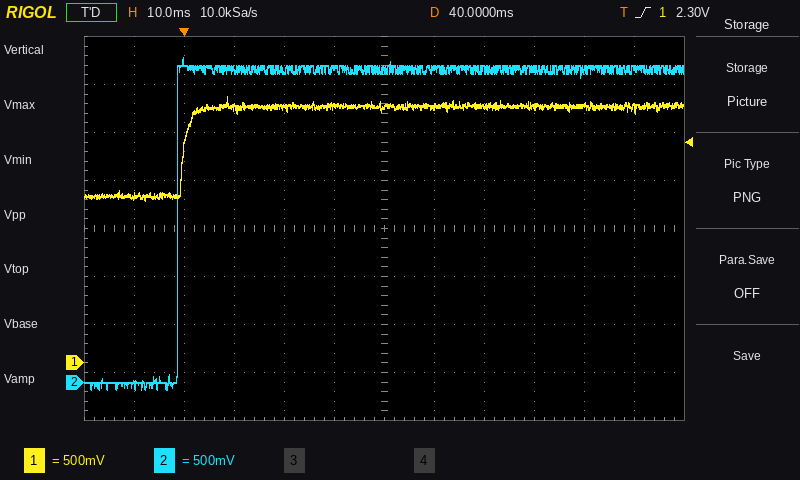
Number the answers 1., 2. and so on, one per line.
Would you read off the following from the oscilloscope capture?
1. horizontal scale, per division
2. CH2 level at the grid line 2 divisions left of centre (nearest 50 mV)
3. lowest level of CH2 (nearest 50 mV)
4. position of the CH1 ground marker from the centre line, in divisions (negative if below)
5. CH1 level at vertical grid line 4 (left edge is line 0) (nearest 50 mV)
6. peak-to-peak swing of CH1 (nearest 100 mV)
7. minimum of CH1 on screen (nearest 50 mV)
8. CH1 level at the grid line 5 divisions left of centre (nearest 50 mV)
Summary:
1. 10 ms
2. 3.25 V
3. -100 mV
4. -2.8 div
5. 2.65 V
6. 1.10 V
7. 1.70 V
8. 1.75 V
